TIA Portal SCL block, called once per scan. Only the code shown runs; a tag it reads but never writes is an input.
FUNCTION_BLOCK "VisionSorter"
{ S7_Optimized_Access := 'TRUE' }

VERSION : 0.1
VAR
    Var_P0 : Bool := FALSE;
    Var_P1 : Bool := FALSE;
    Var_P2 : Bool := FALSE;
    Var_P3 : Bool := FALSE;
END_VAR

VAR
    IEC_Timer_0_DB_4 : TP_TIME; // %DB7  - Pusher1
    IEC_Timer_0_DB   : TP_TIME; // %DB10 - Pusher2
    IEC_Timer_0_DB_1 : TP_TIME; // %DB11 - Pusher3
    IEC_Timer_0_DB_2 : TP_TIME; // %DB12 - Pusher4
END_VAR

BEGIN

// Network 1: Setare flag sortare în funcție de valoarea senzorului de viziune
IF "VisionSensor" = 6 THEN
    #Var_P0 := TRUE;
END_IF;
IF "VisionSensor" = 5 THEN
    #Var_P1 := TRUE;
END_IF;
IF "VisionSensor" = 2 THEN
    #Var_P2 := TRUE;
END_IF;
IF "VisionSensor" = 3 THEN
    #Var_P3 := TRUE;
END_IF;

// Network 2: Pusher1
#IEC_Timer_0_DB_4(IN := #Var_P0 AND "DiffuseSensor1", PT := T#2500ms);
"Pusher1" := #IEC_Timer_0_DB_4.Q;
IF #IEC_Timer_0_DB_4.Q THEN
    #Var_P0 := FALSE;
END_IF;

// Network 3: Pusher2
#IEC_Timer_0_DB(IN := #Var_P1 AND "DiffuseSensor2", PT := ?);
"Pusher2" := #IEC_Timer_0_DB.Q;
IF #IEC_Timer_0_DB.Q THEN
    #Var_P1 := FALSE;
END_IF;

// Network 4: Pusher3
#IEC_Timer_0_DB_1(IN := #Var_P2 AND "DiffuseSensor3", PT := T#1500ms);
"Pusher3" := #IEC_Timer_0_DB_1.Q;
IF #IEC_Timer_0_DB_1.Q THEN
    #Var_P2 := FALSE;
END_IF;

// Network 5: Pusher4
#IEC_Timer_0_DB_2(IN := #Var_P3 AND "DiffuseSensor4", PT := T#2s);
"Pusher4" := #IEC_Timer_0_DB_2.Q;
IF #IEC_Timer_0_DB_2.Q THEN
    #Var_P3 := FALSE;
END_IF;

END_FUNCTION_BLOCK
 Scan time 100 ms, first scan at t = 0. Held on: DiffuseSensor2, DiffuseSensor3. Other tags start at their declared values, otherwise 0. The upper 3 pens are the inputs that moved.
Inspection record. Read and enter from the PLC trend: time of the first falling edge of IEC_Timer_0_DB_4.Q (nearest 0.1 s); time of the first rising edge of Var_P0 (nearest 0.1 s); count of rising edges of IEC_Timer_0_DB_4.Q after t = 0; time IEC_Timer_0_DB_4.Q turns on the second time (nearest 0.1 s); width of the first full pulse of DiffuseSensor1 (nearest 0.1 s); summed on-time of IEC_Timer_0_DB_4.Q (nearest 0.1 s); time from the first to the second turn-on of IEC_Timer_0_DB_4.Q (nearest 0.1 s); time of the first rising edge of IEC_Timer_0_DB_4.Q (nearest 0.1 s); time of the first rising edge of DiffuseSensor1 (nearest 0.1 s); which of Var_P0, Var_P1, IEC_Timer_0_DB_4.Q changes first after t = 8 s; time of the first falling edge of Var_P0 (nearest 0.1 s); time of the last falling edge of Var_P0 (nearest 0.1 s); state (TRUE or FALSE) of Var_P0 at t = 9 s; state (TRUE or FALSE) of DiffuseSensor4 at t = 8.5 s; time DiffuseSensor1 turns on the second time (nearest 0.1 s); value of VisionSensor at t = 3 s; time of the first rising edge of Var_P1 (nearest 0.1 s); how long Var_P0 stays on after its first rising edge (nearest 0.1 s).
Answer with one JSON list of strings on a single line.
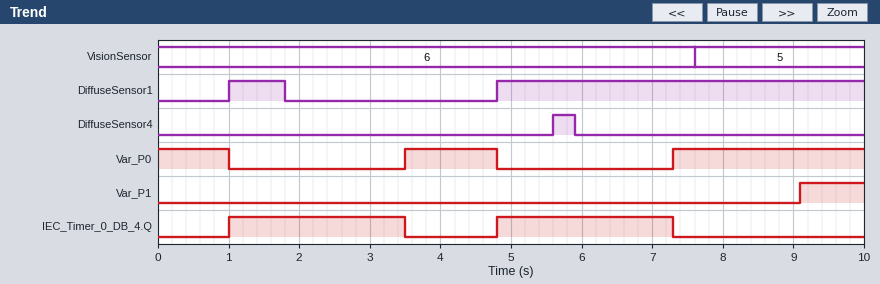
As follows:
["3.5 s", "3.5 s", "2", "4.8 s", "0.8 s", "5.0 s", "3.8 s", "1.0 s", "1.0 s", "Var_P1", "1.0 s", "4.8 s", "TRUE", "FALSE", "4.8 s", "6", "9.1 s", "1.3 s"]
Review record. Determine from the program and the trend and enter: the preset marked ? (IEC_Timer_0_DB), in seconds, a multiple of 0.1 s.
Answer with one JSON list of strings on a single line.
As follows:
["1.5 s"]
